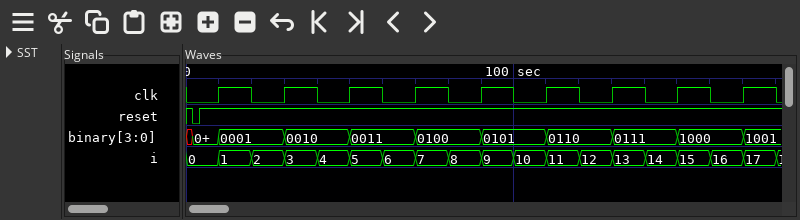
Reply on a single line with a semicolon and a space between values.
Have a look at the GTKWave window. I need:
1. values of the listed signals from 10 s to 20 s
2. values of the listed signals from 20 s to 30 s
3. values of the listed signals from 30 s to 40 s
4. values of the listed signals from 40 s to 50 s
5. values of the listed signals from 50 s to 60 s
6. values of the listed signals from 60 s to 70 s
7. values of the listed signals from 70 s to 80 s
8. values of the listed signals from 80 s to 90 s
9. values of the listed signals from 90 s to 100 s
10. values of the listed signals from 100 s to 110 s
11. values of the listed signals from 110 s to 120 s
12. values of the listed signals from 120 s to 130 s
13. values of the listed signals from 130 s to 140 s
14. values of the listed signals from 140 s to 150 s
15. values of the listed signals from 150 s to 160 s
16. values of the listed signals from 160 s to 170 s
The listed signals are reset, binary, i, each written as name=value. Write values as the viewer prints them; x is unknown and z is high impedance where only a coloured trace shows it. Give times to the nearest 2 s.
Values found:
reset=1, binary=0001, i=1; reset=1, binary=0001, i=2; reset=1, binary=0010, i=3; reset=1, binary=0010, i=4; reset=1, binary=0011, i=5; reset=1, binary=0011, i=6; reset=1, binary=0100, i=7; reset=1, binary=0100, i=8; reset=1, binary=0101, i=9; reset=1, binary=0101, i=10; reset=1, binary=0110, i=11; reset=1, binary=0110, i=12; reset=1, binary=0111, i=13; reset=1, binary=0111, i=14; reset=1, binary=1000, i=15; reset=1, binary=1000, i=16
